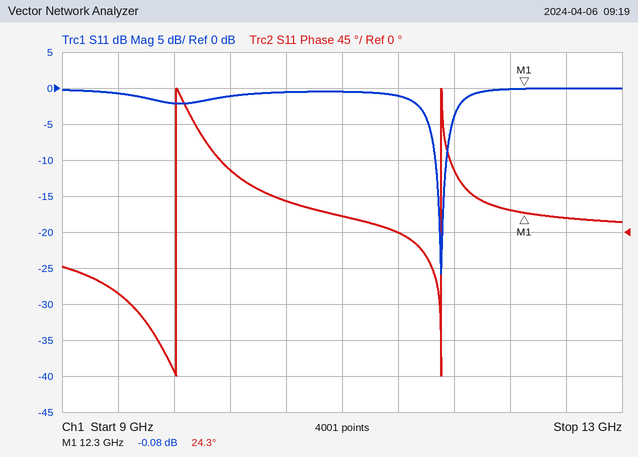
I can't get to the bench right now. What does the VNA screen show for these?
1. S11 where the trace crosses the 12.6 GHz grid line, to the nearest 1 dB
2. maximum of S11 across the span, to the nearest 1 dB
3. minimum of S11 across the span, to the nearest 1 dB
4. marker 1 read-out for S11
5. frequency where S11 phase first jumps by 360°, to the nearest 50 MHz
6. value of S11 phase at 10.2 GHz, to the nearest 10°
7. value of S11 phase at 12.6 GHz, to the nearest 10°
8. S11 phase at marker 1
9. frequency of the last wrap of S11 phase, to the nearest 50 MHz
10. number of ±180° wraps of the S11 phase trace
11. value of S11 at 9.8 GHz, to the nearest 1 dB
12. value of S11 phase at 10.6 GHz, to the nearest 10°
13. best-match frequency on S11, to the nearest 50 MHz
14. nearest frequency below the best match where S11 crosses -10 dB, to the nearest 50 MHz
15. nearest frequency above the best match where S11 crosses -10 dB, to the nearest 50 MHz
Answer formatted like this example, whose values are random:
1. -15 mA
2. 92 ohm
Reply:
1. 0 dB
2. 0 dB
3. -26 dB
4. -0.08 dB
5. 9.80 GHz
6. 80°
7. 20°
8. 24.3°
9. 11.70 GHz
10. 2
11. -2 dB
12. 40°
13. 11.70 GHz
14. 11.65 GHz
15. 11.75 GHz
